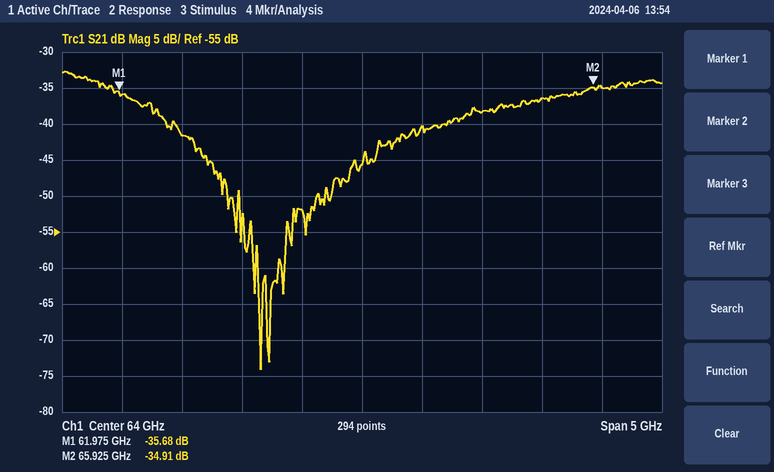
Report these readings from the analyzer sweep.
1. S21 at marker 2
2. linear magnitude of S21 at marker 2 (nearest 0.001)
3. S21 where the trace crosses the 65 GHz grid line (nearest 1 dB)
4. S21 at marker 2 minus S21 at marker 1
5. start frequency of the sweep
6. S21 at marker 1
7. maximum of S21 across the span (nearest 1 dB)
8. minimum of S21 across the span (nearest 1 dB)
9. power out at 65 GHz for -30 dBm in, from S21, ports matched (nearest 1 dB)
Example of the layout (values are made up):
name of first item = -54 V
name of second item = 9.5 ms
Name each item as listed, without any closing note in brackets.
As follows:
S21 at marker 2 = -34.91 dB
linear magnitude of S21 at marker 2 = 0.018
S21 where the trace crosses the 65 GHz grid line = -38 dB
S21 at marker 2 minus S21 at marker 1 = 0.77 dB
start frequency of the sweep = 61.5 GHz
S21 at marker 1 = -35.68 dB
maximum of S21 across the span = -33 dB
minimum of S21 across the span = -74 dB
power out at 65 GHz for -30 dBm in, from S21, ports matched = -68 dBm
